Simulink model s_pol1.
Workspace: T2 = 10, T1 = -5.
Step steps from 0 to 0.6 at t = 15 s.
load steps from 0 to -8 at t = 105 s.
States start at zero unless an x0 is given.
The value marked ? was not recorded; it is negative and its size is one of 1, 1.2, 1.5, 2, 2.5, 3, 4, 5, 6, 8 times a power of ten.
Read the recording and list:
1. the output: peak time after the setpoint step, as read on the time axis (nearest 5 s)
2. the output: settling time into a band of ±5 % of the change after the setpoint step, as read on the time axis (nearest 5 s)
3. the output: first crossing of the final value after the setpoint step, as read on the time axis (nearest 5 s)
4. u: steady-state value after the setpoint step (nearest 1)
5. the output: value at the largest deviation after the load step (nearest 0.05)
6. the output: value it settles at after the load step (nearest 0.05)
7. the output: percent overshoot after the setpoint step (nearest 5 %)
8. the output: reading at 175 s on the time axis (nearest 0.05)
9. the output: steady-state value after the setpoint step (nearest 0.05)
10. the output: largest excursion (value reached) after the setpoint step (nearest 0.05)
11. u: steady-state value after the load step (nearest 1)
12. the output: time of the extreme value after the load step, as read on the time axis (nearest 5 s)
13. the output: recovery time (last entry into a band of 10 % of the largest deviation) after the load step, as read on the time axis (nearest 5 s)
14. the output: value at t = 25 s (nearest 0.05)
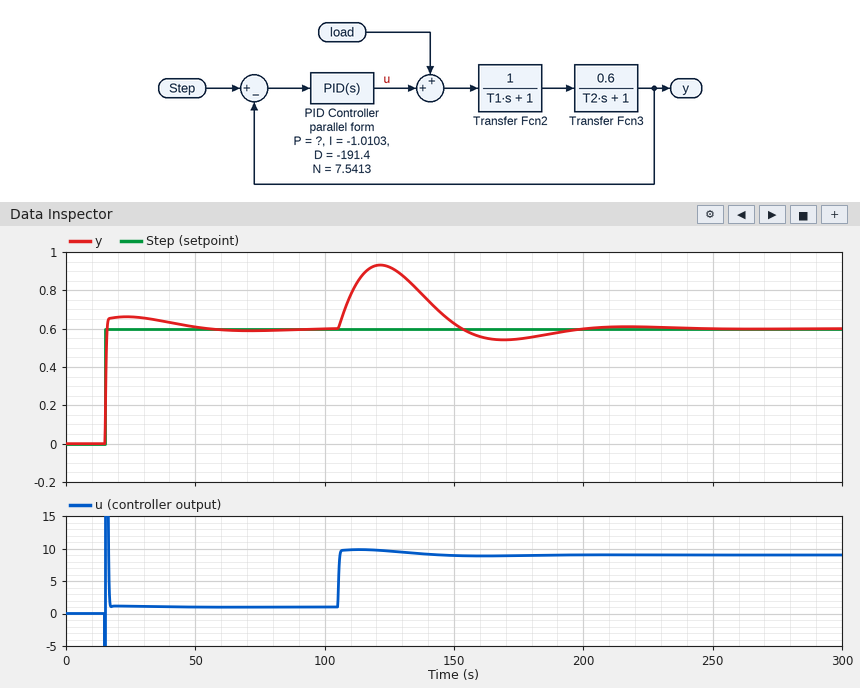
25 s
40 s
15 s
1
0.95
0.60
10 %
0.55
0.60
0.65
9
120 s
185 s
0.65
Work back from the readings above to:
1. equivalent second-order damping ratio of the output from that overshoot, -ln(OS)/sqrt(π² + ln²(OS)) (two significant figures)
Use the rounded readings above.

0.59
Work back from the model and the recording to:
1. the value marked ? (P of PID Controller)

-15
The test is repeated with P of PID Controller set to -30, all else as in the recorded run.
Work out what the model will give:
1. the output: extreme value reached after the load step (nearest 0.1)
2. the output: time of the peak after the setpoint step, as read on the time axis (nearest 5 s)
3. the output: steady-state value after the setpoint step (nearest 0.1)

0.8
15 s
0.6
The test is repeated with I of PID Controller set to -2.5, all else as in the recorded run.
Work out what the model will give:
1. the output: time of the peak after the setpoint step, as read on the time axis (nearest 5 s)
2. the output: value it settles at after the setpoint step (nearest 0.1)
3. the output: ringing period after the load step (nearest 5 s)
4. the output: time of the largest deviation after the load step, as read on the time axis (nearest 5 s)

20 s
0.6
55 s
115 s
